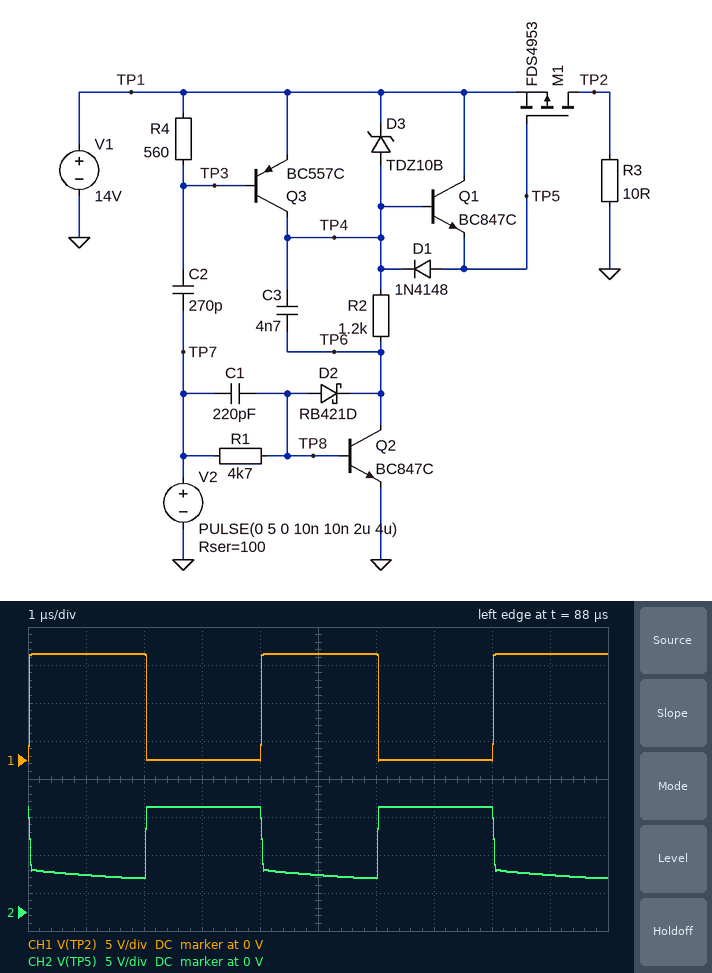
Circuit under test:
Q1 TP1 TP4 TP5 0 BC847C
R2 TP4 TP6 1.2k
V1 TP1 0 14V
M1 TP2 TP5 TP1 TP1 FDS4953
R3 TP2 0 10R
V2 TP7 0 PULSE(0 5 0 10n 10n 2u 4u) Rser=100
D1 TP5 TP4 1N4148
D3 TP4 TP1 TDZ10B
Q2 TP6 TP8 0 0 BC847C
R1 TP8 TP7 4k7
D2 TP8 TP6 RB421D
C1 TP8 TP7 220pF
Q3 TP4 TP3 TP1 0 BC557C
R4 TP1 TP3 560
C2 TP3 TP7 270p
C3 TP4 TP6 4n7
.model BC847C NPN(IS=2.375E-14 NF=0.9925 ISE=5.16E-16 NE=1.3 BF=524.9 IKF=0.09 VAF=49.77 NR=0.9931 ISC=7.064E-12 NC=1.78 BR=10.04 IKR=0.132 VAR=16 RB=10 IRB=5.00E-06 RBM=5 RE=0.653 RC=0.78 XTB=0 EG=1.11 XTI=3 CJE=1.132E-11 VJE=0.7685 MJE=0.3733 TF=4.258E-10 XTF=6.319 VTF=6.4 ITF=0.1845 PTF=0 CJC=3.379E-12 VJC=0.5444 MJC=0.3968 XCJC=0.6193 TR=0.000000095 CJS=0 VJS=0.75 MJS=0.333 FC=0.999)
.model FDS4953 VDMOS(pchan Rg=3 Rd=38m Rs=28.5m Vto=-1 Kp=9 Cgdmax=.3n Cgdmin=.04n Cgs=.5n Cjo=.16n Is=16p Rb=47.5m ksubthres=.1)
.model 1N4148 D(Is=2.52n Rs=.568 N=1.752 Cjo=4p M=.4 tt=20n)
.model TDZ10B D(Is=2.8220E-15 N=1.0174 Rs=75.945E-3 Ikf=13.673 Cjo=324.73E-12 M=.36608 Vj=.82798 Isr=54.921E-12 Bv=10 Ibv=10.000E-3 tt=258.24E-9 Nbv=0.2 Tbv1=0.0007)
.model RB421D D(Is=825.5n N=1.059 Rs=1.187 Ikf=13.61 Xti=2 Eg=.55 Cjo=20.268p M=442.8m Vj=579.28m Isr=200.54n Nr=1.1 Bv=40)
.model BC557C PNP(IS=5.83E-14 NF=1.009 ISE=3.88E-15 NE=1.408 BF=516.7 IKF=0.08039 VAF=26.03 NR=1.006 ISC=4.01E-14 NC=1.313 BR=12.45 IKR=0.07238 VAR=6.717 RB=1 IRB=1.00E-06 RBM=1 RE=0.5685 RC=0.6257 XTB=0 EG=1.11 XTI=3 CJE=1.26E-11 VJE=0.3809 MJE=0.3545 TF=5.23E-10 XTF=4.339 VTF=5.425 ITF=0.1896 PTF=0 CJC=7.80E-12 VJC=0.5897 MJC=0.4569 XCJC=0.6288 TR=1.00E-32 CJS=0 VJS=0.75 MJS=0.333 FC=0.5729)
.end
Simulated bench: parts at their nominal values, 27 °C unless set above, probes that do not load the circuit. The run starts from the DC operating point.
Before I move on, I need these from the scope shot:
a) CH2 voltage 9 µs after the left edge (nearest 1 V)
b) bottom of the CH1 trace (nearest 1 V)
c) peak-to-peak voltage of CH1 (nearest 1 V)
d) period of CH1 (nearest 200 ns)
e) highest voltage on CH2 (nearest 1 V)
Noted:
5 V
0 V
14 V
4.0 µs
14 V
